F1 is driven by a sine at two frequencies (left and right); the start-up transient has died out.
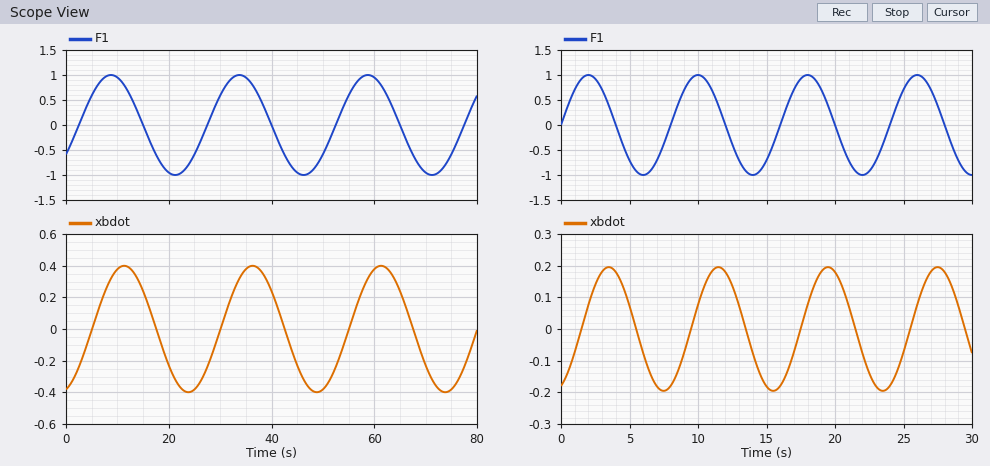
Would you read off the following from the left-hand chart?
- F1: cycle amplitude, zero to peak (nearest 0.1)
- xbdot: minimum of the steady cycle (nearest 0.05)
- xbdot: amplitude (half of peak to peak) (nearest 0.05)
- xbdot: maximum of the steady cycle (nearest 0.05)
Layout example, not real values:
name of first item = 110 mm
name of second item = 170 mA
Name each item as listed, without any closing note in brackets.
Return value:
F1: cycle amplitude, zero to peak = 1.0
xbdot: minimum of the steady cycle = -0.40
xbdot: amplitude (half of peak to peak) = 0.40
xbdot: maximum of the steady cycle = 0.40
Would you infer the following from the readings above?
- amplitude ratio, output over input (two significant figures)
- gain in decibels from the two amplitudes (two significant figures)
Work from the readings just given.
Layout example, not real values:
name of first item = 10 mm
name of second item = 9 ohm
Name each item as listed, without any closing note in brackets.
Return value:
amplitude ratio, output over input = 0.40
gain in decibels from the two amplitudes = -8.0 dB
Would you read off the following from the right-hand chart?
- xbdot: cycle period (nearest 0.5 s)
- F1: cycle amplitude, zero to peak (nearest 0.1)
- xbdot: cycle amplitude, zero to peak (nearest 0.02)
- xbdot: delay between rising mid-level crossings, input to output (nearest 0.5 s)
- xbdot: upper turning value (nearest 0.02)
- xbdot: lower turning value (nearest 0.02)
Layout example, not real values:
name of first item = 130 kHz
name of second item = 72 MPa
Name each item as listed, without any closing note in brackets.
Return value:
xbdot: cycle period = 8.0 s
F1: cycle amplitude, zero to peak = 1.0
xbdot: cycle amplitude, zero to peak = 0.20
xbdot: delay between rising mid-level crossings, input to output = 1.5 s
xbdot: upper turning value = 0.20
xbdot: lower turning value = -0.20
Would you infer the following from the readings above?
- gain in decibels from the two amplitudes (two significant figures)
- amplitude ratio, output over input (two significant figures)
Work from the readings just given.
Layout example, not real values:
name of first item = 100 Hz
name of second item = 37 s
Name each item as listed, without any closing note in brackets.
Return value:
gain in decibels from the two amplitudes = -14 dB
amplitude ratio, output over input = 0.20
